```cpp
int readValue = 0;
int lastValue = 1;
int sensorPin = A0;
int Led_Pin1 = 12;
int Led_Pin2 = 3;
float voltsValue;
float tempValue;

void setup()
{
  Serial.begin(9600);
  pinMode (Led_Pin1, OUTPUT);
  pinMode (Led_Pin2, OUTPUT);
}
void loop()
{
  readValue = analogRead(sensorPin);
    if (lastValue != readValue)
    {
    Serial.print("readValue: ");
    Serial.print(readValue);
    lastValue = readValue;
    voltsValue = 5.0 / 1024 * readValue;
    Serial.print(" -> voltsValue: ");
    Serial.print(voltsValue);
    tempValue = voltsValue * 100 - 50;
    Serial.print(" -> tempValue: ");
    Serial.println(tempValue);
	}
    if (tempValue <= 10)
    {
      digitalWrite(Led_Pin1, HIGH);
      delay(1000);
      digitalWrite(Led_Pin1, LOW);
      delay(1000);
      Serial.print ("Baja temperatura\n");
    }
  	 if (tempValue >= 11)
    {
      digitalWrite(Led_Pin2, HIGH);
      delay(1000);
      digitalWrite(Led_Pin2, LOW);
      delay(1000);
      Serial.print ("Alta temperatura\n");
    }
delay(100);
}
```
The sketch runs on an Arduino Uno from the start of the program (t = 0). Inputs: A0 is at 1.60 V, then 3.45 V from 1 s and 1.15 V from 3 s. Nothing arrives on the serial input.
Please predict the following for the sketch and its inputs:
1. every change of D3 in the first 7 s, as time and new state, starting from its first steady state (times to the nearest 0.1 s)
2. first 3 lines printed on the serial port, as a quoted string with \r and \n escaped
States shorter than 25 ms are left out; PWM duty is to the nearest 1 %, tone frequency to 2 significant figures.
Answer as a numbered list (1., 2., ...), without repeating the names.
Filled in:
1. 0 s high; 1 s low; 2.1 s high; 3.1 s low; 4.2 s high; 5.2 s low; 6.3 s high
2. "readValue: 327 -> voltsValue: 1.60 -> tempValue: 109.67\r\nAlta temperatura\nreadValue: 706 -> voltsValue: 3.45 -> tempValue: 294.73\r\n"
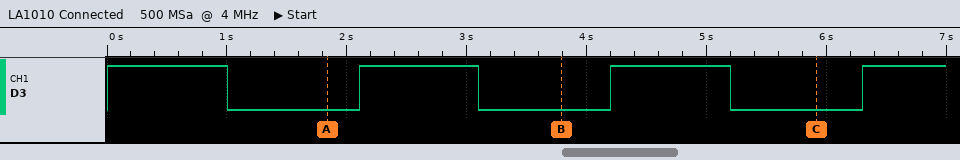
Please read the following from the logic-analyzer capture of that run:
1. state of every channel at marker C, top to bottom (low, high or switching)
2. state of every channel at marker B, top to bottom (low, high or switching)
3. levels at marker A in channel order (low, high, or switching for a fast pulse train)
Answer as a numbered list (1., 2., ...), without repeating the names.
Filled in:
1. D3 low
2. D3 low
3. D3 low
